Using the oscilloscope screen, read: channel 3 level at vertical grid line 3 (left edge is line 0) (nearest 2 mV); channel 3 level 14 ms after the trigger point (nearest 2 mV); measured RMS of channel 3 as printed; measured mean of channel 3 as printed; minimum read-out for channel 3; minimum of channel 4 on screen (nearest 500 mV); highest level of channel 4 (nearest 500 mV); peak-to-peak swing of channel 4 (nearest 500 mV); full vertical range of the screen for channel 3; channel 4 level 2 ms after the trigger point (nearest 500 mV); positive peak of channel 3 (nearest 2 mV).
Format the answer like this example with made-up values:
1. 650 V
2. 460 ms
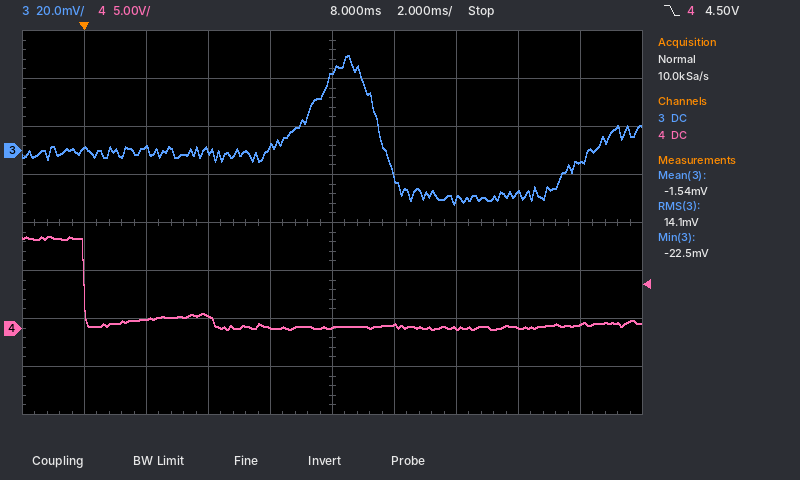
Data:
1. 0 mV
2. -18 mV
3. 14.1 mV
4. -1.54 mV
5. -22.5 mV
6. 0.0 V
7. 9.5 V
8. 9.5 V
9. 160 mV
10. 1.0 V
11. 40 mV
